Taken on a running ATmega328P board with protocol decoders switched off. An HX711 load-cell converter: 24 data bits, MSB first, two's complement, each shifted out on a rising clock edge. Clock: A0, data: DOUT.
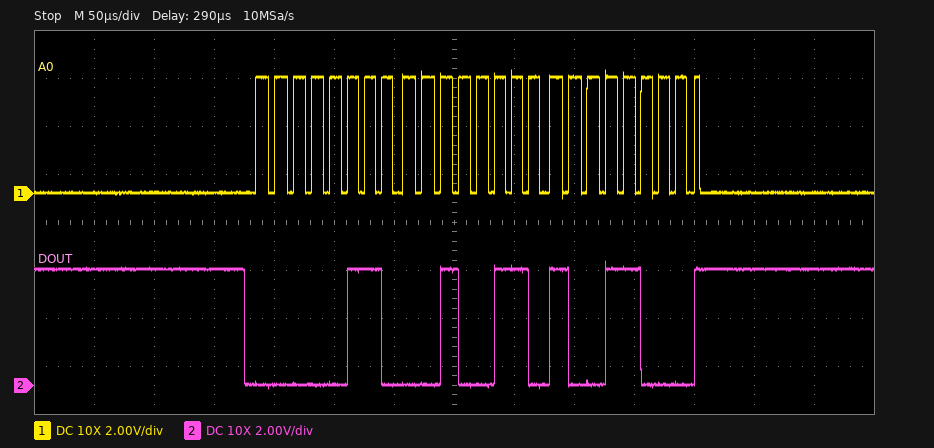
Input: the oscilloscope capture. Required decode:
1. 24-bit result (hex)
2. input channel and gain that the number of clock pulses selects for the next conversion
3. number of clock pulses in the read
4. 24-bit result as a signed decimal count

0x062698
channel A, gain 128
25
403096
